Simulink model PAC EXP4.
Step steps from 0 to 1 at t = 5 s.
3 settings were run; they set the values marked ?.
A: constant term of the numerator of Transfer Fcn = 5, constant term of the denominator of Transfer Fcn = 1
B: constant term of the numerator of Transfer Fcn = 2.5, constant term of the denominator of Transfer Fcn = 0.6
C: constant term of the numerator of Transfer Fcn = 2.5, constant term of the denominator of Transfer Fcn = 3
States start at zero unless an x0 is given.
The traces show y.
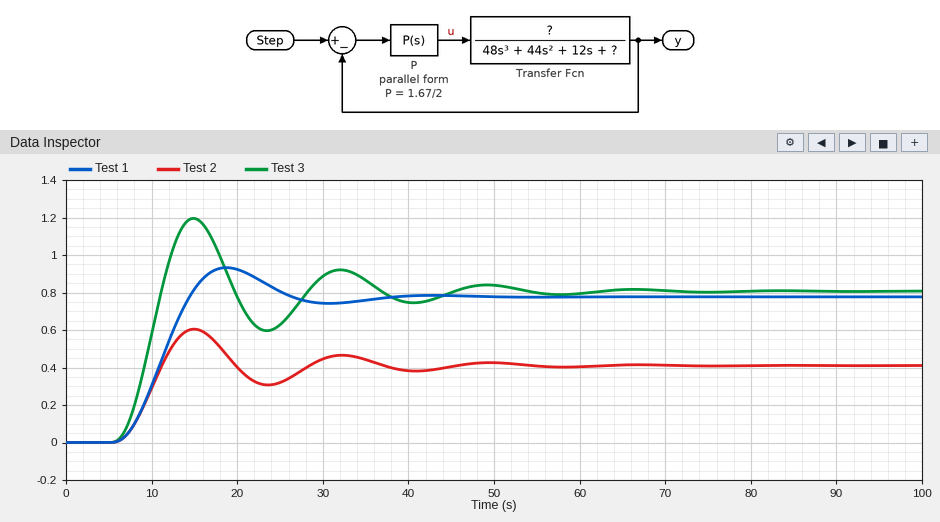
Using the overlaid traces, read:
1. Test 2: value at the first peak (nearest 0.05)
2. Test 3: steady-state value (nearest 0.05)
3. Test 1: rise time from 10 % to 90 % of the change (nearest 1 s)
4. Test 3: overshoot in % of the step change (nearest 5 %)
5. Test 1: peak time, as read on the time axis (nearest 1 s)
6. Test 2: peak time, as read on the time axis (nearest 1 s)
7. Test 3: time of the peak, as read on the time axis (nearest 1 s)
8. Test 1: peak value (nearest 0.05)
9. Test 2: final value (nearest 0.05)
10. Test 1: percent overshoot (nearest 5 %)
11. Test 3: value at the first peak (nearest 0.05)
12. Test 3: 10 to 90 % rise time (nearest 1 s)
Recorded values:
0.60
0.80
6 s
50 %
19 s
15 s
15 s
0.95
0.40
20 %
1.20
4 s
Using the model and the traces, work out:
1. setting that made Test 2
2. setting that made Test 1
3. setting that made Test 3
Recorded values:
C
B
A
